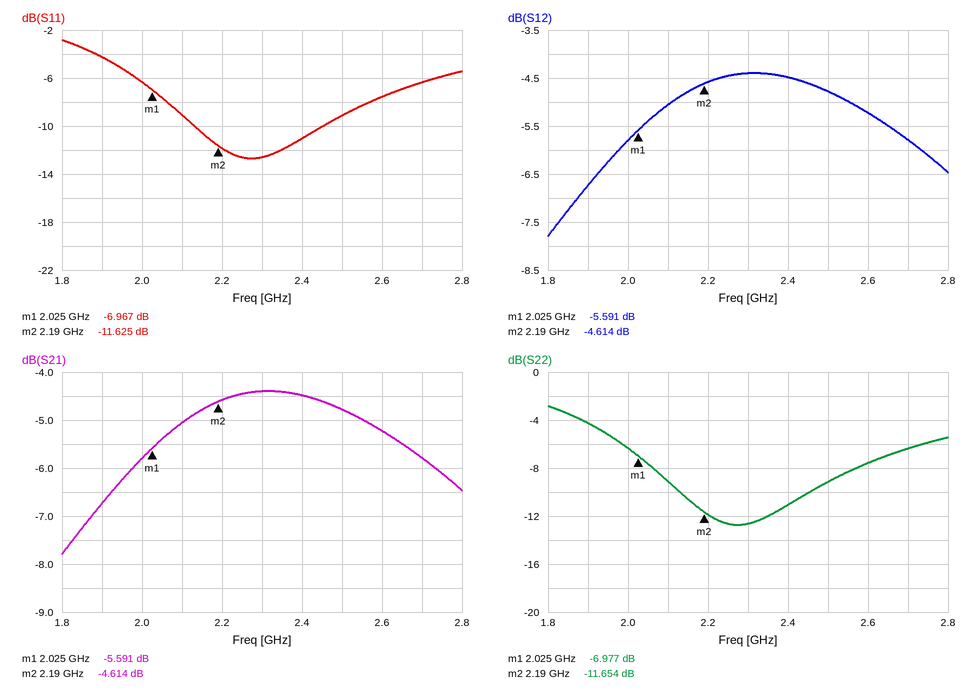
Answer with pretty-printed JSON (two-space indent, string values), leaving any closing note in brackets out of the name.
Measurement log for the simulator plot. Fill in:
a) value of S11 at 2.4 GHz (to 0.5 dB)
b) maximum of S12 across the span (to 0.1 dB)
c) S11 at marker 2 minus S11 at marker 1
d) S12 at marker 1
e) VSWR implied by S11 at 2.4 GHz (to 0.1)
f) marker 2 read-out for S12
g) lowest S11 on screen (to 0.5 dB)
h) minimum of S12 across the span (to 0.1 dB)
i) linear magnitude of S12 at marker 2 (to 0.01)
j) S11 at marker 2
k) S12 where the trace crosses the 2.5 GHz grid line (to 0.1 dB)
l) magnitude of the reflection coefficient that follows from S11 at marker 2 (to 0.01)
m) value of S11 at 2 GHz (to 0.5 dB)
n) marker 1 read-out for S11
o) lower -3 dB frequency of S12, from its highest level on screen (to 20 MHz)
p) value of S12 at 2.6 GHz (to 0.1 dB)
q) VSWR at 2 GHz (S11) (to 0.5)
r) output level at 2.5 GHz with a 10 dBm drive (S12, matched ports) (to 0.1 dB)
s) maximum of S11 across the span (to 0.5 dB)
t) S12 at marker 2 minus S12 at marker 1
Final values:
{
  "value of S11 at 2.4 GHz": "-11.0 dB",
  "maximum of S12 across the span": "-4.4 dB",
  "S11 at marker 2 minus S11 at marker 1": "-4.658 dB",
  "S12 at marker 1": "-5.591 dB",
  "VSWR implied by S11 at 2.4 GHz": "1.8",
  "marker 2 read-out for S12": "-4.614 dB",
  "lowest S11 on screen": "-12.5 dB",
  "minimum of S12 across the span": "-7.8 dB",
  "linear magnitude of S12 at marker 2": "0.59",
  "S11 at marker 2": "-11.625 dB",
  "S12 where the trace crosses the 2.5 GHz grid line": "-4.8 dB",
  "magnitude of the reflection coefficient that follows from S11 at marker 2": "0.26",
  "value of S11 at 2 GHz": "-6.5 dB",
  "marker 1 read-out for S11": "-6.967 dB",
  "lower -3 dB frequency of S12, from its highest level on screen": "1.84 GHz",
  "value of S12 at 2.6 GHz": "-5.2 dB",
  "VSWR at 2 GHz (S11)": "3.0",
  "output level at 2.5 GHz with a 10 dBm drive (S12, matched ports)": "5.2 dBm",
  "maximum of S11 across the span": "-3.0 dB",
  "S12 at marker 2 minus S12 at marker 1": "0.977 dB"
}
